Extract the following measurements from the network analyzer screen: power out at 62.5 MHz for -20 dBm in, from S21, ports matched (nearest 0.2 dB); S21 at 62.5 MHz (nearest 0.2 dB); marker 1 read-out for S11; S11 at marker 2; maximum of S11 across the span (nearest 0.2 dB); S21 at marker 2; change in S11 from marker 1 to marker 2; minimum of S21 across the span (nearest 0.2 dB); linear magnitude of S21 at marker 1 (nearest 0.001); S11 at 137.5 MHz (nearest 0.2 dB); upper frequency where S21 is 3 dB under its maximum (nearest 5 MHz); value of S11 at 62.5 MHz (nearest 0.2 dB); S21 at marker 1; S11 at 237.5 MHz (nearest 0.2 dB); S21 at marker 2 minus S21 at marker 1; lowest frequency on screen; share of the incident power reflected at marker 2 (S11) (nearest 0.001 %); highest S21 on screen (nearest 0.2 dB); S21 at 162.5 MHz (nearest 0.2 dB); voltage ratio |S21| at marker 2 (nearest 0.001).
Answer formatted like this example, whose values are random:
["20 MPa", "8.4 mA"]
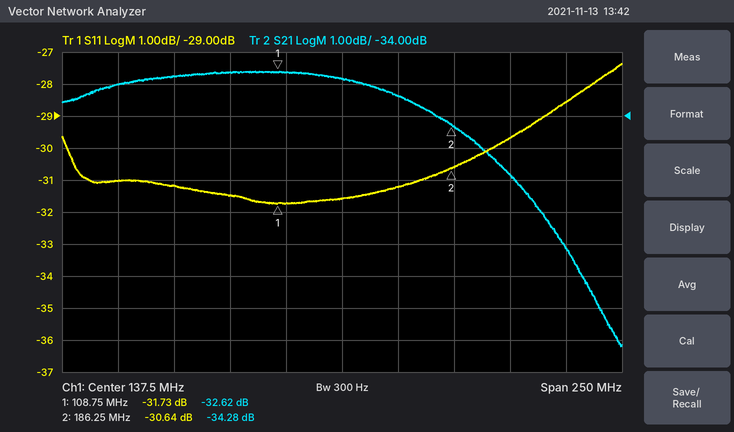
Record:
["-52.8 dBm", "-32.8 dB", "-31.73 dB", "-30.64 dB", "-27.4 dB", "-34.28 dB", "1.09 dB", "-41.2 dB", "0.023", "-31.6 dB", "210 MHz", "-31.2 dB", "-32.62 dB", "-28.6 dB", "-1.66 dB", "12.5 MHz", "0.086 %", "-32.6 dB", "-33.4 dB", "0.019"]
